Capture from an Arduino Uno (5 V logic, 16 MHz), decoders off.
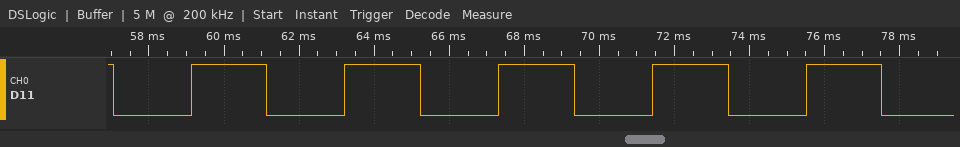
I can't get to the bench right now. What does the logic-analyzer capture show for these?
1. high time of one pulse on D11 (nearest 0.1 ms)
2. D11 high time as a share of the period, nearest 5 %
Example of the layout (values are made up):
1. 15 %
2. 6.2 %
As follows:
1. 2.0 ms
2. 50 %
